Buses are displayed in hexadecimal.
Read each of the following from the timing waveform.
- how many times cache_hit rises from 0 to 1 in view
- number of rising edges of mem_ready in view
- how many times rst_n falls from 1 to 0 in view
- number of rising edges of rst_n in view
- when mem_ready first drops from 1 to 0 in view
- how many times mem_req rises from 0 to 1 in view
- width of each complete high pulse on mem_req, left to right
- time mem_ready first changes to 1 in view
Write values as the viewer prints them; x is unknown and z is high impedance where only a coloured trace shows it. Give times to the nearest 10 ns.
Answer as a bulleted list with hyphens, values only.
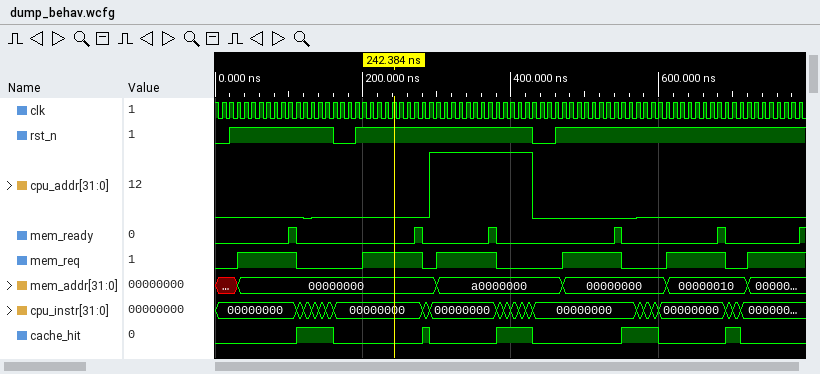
- 5
- 6
- 2
- 3
- 110 ns
- 6
- 80 ns, 80 ns, 80 ns, 80 ns, 80 ns
- 100 ns
